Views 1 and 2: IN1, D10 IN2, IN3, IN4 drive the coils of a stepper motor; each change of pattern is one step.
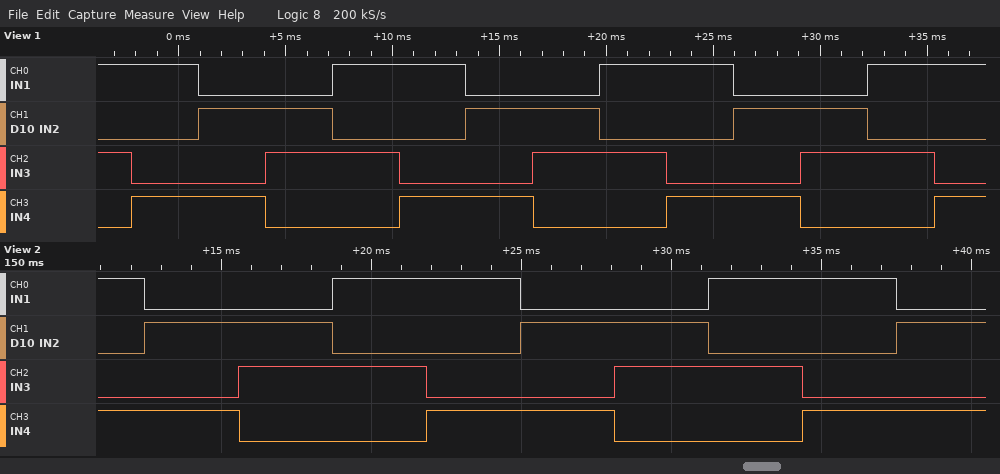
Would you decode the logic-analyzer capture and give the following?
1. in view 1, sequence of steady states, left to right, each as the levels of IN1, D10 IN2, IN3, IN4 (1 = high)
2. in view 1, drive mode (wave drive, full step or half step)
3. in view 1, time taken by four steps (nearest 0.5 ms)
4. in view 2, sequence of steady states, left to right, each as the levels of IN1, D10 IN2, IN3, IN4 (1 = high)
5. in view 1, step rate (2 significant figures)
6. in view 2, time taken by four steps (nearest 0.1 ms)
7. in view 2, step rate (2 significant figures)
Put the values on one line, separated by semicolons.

1010 1001 0101 0110 1010 1001 0101 0110 1010 1001 0101 0110 1010 1001; full step; 12.5 ms; 1001 0101 0110 1010 1001 0101 0110 1010 1001 0101; 320 steps/s; 12.5 ms; 320 steps/s
